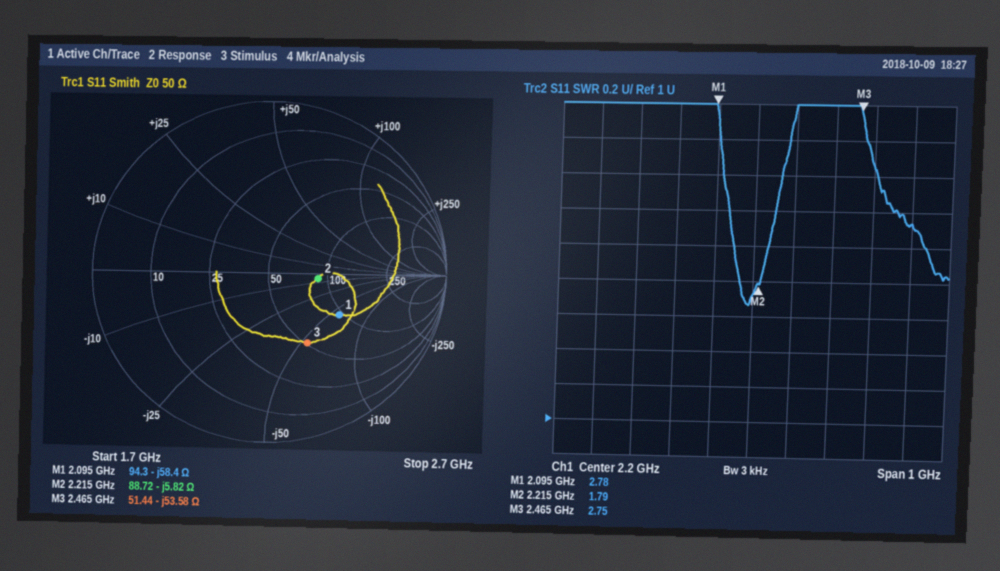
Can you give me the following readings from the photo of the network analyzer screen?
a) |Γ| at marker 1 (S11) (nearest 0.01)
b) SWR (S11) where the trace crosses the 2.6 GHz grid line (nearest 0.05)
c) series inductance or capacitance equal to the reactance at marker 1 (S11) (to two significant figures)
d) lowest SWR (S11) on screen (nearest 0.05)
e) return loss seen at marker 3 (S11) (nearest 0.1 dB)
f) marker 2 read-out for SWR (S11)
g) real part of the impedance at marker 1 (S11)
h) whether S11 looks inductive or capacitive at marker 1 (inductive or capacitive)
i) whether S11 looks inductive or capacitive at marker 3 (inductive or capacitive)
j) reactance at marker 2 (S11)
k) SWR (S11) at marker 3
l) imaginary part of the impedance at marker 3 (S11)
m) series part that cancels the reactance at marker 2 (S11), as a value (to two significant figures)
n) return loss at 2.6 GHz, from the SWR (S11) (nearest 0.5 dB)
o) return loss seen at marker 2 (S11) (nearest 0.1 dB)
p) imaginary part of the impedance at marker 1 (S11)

0.47
2.15
1.3 pF
1.65
6.6 dB
1.79
94.3 Ω
capacitive
capacitive
-5.82 Ω
2.75
-53.58 Ω
420 pH
9.0 dB
11.0 dB
-58.4 Ω
